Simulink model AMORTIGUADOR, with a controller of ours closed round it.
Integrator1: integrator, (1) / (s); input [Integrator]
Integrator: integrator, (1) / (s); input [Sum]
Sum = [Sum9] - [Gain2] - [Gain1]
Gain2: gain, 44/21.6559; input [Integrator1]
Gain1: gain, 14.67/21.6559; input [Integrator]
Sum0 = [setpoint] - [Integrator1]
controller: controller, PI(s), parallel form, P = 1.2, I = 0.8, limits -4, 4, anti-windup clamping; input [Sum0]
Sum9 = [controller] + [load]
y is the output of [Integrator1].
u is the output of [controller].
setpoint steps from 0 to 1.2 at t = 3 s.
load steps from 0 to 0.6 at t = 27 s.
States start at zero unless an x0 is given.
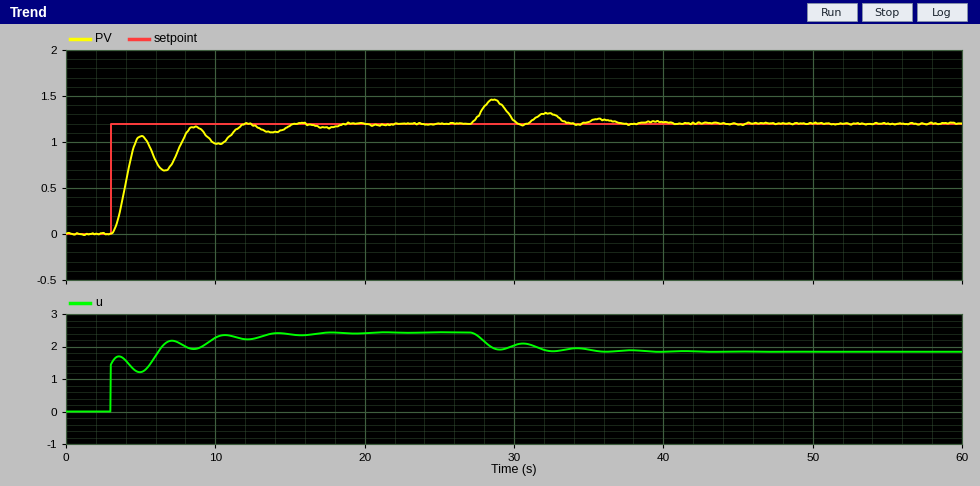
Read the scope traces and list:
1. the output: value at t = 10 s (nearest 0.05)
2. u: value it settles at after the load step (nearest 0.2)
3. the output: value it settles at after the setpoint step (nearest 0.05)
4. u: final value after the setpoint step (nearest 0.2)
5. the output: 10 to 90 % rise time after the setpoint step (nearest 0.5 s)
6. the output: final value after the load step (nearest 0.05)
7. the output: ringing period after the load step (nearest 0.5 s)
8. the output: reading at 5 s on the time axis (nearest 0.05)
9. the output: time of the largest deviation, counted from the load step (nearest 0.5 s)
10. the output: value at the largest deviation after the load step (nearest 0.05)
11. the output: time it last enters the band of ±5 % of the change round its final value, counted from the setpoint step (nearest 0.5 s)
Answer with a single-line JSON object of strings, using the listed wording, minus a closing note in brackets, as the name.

{"the output: value at t = 10 s": "1.00", "u: value it settles at after the load step": "1.8", "the output: value it settles at after the setpoint step": "1.20", "u: final value after the setpoint step": "2.4", "the output: 10 to 90 % rise time after the setpoint step": "4.5 s", "the output: final value after the load step": "1.20", "the output: ringing period after the load step": "3.5 s", "the output: reading at 5 s on the time axis": "1.05", "the output: time of the largest deviation, counted from the load step": "1.5 s", "the output: value at the largest deviation after the load step": "1.45", "the output: time it last enters the band of ±5 % of the change round its final value, counted from the setpoint step": "11.5 s"}
